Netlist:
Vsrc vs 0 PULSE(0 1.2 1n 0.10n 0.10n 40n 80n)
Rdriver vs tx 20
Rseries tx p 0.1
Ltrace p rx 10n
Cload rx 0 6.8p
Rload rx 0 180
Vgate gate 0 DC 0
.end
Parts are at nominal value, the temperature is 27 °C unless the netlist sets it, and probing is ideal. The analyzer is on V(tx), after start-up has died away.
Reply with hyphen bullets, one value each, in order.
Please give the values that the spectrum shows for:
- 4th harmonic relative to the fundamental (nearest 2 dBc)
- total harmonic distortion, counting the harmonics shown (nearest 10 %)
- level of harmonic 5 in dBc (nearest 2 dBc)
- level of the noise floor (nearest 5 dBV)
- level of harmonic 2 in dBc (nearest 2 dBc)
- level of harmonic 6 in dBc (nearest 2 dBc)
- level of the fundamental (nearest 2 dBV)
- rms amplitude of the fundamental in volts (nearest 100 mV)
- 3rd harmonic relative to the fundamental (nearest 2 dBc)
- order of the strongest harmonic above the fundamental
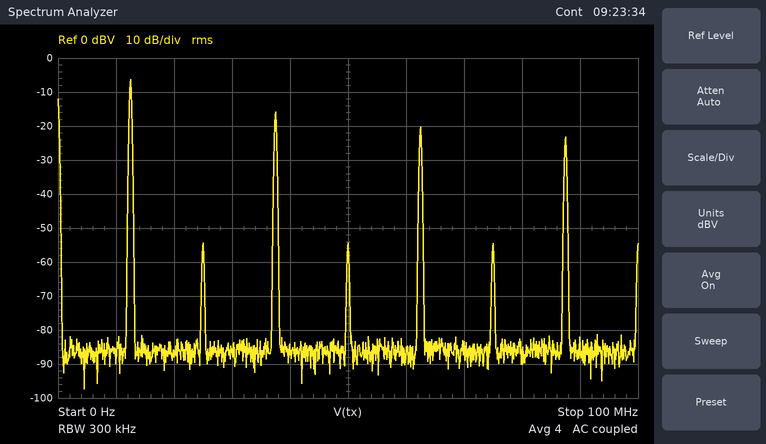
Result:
- -48 dBc
- 40 %
- -14 dBc
- -85 dBV
- -48 dBc
- -48 dBc
- -6 dBV
- 500 mV
- -10 dBc
- 3
